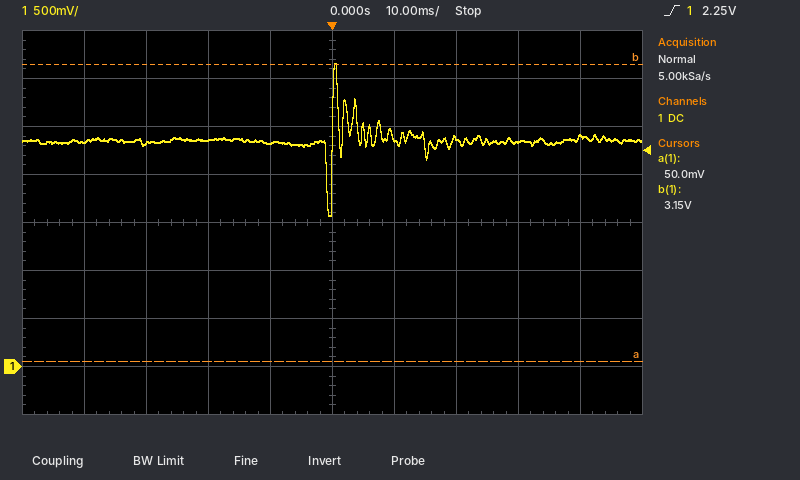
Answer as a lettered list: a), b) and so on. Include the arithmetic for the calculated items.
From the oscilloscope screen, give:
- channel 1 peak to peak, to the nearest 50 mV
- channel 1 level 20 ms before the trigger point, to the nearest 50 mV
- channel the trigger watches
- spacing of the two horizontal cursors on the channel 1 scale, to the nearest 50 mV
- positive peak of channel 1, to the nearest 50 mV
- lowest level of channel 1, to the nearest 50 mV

a) 3.15 V − (1.55 V) = 1.60 V
b) 2.35 V
c) channel 1
d) 3.10 V
e) 3.15 V
f) 1.55 V
